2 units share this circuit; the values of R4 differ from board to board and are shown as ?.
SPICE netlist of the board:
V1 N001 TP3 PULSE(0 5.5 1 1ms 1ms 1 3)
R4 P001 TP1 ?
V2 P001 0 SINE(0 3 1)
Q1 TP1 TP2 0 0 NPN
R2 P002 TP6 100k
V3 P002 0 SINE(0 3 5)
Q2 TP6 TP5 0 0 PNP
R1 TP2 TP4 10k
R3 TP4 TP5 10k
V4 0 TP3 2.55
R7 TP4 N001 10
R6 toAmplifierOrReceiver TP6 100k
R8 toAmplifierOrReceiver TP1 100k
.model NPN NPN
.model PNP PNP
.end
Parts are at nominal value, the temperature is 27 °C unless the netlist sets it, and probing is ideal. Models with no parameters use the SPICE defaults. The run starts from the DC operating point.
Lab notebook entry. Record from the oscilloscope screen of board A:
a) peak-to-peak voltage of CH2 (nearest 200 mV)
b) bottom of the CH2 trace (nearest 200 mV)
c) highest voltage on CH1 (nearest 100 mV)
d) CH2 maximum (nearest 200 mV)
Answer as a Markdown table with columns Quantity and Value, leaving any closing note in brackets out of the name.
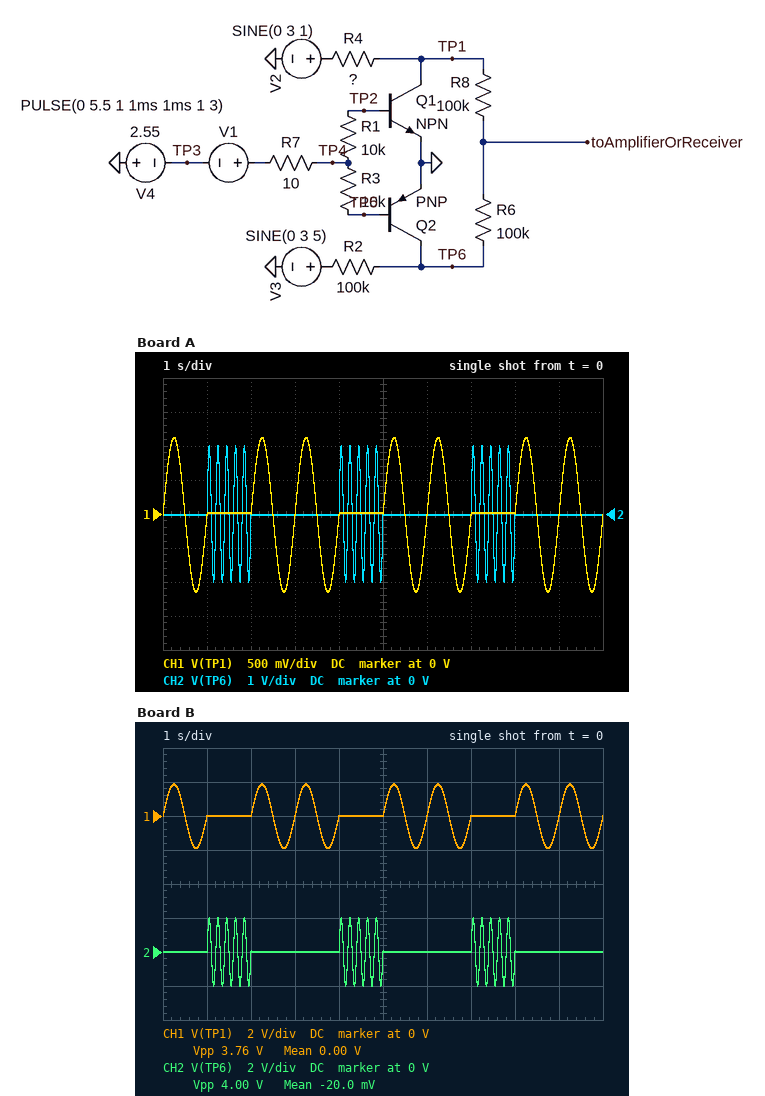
| Quantity | Value |
|---|---|
| peak-to-peak voltage of CH2 | 4.0 V |
| bottom of the CH2 trace | -2.0 V |
| highest voltage on CH1 | 1.1 V |
| CH2 maximum | 2.0 V |
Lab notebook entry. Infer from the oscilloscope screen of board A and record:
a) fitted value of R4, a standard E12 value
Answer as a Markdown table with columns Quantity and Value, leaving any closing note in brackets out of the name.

| Quantity | Value |
|---|---|
| fitted value of R4, a standard E12 value | 330 kΩ |
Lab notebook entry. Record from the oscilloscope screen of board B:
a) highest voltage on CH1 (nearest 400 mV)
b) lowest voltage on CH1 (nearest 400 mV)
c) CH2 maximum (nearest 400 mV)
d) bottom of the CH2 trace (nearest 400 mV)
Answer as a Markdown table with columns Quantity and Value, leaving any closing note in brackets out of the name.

| Quantity | Value |
|---|---|
| highest voltage on CH1 | 2.0 V |
| lowest voltage on CH1 | -2.0 V |
| CH2 maximum | 2.0 V |
| bottom of the CH2 trace | -2.0 V |
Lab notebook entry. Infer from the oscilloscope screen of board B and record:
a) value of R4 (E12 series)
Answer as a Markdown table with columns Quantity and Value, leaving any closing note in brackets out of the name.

| Quantity | Value |
|---|---|
| value of R4 | 120 kΩ |
